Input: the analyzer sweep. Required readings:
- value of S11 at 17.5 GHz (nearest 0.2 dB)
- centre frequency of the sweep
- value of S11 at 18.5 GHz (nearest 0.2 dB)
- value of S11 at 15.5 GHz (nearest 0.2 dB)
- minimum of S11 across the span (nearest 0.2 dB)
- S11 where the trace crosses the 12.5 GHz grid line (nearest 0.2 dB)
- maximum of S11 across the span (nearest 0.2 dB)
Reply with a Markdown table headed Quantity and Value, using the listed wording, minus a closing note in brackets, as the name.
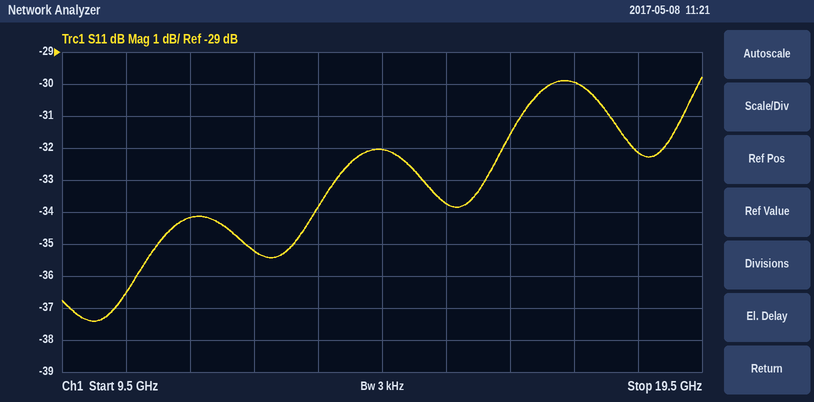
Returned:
| Quantity | Value |
|---|---|
| value of S11 at 17.5 GHz | -30.0 dB |
| centre frequency of the sweep | 14.5 GHz |
| value of S11 at 18.5 GHz | -32.2 dB |
| value of S11 at 15.5 GHz | -33.8 dB |
| minimum of S11 across the span | -37.4 dB |
| S11 where the trace crosses the 12.5 GHz grid line | -35.2 dB |
| maximum of S11 across the span | -29.8 dB |
